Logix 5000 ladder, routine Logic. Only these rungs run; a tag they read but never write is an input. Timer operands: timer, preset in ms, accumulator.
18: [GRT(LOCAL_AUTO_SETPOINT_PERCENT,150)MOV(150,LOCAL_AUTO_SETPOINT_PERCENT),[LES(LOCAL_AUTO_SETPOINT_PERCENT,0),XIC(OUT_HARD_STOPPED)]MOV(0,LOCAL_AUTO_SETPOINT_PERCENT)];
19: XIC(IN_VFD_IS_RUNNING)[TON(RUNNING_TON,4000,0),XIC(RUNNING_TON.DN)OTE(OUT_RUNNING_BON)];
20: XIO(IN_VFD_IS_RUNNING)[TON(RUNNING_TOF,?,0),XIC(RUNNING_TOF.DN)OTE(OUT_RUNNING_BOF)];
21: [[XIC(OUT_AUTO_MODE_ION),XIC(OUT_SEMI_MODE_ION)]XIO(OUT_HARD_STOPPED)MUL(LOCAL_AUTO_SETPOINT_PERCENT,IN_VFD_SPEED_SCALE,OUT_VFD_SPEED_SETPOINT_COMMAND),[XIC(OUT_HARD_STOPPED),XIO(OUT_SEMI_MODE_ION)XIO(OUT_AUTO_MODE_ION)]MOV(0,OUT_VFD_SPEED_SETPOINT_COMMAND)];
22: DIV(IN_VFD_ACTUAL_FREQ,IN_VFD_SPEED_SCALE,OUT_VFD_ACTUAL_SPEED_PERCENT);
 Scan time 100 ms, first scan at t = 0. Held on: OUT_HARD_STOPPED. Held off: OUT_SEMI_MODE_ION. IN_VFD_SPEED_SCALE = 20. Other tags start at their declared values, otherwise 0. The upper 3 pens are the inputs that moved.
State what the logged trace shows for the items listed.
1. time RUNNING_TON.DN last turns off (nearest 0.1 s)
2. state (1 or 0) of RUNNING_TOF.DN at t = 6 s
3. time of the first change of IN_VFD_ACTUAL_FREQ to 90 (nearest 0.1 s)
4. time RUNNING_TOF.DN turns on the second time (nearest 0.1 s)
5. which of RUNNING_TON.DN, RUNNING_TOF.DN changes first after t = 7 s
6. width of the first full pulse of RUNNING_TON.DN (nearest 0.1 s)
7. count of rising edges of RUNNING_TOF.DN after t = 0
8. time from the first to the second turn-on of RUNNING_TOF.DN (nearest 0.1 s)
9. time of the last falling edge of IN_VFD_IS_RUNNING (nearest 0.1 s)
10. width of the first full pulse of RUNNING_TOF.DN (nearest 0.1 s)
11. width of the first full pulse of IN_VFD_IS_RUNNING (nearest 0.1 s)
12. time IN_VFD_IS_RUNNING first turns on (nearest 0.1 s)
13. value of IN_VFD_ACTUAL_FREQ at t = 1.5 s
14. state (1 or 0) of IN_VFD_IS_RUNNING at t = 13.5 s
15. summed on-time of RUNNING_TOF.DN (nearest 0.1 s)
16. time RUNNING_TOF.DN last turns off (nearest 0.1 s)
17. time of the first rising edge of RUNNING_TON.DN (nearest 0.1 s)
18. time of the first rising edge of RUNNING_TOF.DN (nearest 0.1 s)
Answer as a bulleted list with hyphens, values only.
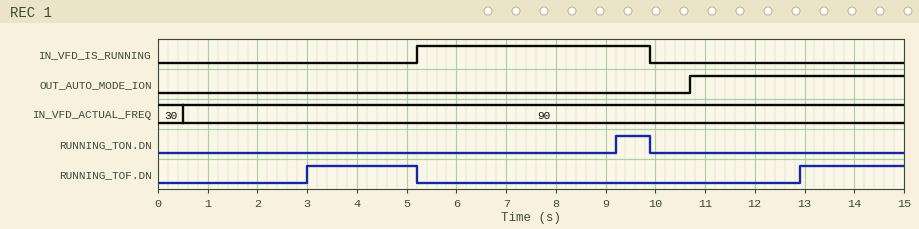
- 9.9 s
- 0
- 0.5 s
- 12.9 s
- RUNNING_TON.DN
- 0.7 s
- 2
- 9.9 s
- 9.9 s
- 2.2 s
- 4.7 s
- 5.2 s
- 90
- 0
- 4.3 s
- 5.2 s
- 9.2 s
- 3.0 s
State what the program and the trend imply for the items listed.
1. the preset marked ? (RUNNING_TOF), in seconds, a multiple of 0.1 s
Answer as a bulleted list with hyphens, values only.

- 3.0 s
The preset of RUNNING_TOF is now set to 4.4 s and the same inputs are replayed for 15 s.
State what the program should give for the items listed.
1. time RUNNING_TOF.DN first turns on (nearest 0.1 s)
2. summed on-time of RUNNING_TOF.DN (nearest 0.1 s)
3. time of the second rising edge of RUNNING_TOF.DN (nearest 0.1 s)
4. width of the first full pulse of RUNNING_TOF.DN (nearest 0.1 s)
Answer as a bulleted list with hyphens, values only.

- 4.4 s
- 1.5 s
- 14.3 s
- 0.8 s
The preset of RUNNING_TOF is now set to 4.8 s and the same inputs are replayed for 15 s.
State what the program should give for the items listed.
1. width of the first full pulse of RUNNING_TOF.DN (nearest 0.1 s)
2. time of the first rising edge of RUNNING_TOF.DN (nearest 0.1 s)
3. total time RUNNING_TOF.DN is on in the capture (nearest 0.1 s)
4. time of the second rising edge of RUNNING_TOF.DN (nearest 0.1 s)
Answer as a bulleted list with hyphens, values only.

- 0.4 s
- 4.8 s
- 0.7 s
- 14.7 s
